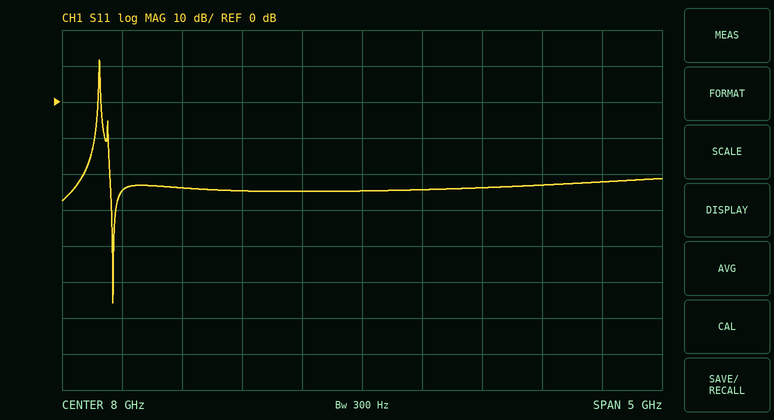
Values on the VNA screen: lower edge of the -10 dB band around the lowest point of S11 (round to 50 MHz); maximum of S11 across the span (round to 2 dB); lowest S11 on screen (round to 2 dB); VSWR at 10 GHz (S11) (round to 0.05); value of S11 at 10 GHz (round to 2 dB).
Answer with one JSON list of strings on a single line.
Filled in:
["5.90 GHz", "12 dB", "-56 dB", "1.15", "-22 dB"]
